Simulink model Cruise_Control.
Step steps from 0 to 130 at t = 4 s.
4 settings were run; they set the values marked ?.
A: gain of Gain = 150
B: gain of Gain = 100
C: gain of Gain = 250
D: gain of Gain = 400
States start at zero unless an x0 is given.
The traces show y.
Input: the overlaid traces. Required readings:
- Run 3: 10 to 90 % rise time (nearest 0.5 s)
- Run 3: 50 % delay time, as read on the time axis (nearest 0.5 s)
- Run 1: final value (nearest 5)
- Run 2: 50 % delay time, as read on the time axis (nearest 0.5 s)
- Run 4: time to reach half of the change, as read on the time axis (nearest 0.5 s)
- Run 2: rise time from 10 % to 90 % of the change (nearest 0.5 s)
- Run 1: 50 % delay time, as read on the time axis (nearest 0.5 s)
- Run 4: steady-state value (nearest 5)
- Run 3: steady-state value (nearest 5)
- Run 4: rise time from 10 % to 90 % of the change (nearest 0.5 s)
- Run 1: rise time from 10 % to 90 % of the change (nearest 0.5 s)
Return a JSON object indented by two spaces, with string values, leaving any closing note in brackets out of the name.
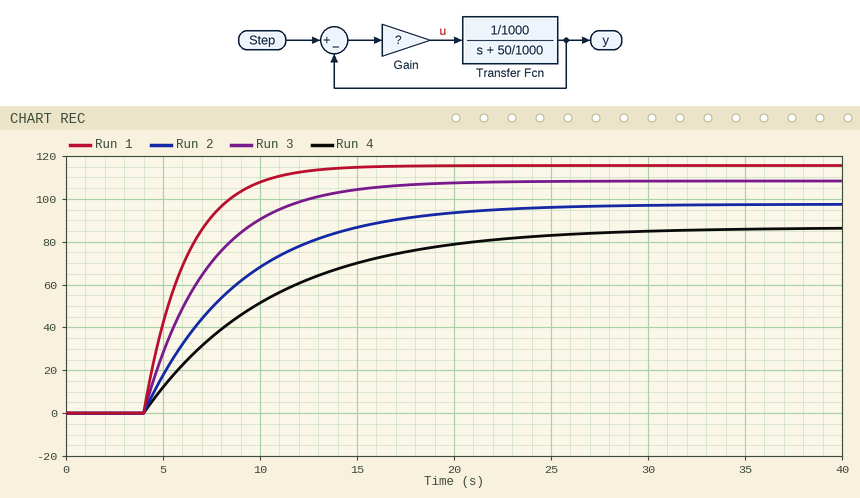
{
  "Run 3: 10 to 90 % rise time": "7.5 s",
  "Run 3: 50 % delay time, as read on the time axis": "6.5 s",
  "Run 1: final value": "115",
  "Run 2: 50 % delay time, as read on the time axis": "7.5 s",
  "Run 4: time to reach half of the change, as read on the time axis": "8.5 s",
  "Run 2: rise time from 10 % to 90 % of the change": "11.0 s",
  "Run 1: 50 % delay time, as read on the time axis": "5.5 s",
  "Run 4: steady-state value": "85",
  "Run 3: steady-state value": "110",
  "Run 4: rise time from 10 % to 90 % of the change": "14.5 s",
  "Run 1: rise time from 10 % to 90 % of the change": "5.0 s"
}
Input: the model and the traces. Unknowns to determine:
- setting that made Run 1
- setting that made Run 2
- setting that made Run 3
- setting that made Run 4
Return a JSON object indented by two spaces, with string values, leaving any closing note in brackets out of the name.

{
  "setting that made Run 1": "D",
  "setting that made Run 2": "A",
  "setting that made Run 3": "C",
  "setting that made Run 4": "B"
}
